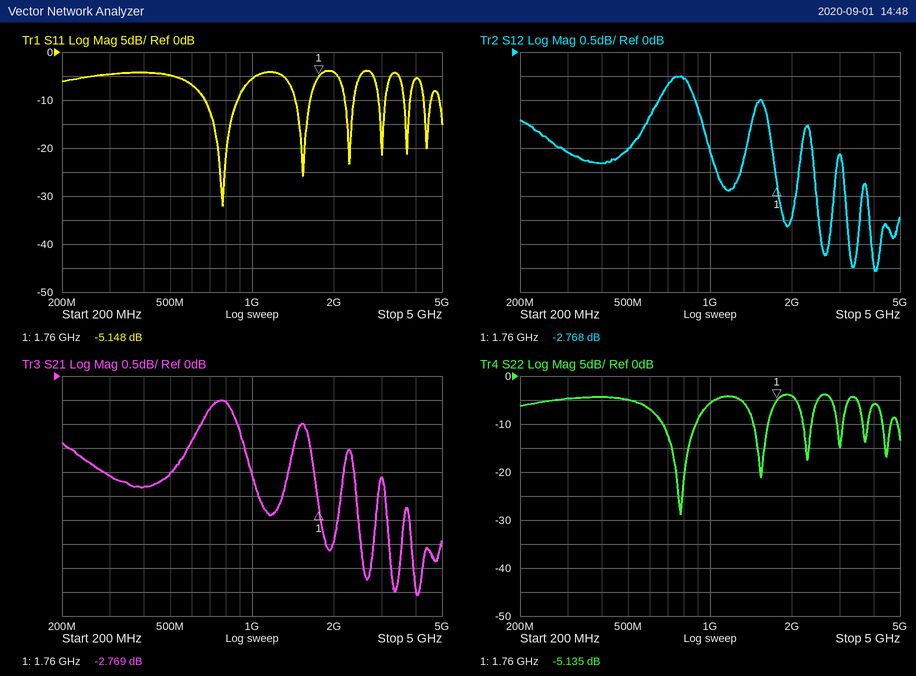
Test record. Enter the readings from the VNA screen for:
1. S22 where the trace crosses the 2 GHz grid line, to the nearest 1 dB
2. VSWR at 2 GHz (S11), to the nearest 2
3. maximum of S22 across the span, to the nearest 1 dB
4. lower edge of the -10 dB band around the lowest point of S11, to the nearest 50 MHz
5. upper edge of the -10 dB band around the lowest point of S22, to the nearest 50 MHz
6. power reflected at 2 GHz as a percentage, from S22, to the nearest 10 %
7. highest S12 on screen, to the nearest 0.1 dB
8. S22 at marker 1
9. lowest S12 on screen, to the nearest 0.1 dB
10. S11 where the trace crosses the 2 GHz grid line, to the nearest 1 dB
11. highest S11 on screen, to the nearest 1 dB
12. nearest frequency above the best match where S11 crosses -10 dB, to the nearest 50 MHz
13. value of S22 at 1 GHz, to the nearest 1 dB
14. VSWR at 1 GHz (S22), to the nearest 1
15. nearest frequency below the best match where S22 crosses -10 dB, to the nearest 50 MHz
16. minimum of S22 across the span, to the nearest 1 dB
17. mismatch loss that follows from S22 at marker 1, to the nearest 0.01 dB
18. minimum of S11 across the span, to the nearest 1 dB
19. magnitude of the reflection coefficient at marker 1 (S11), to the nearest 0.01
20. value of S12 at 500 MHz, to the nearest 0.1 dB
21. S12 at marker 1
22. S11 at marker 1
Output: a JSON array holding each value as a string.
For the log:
["-4 dB", "4", "-4 dB", "650 MHz", "900 MHz", "40 %", "-0.5 dB", "-5.135 dB", "-4.6 dB", "-4 dB", "-4 dB", "900 MHz", "-6 dB", "3", "650 MHz", "-29 dB", "1.59 dB", "-32 dB", "0.55", "-2.0 dB", "-2.768 dB", "-5.148 dB"]
